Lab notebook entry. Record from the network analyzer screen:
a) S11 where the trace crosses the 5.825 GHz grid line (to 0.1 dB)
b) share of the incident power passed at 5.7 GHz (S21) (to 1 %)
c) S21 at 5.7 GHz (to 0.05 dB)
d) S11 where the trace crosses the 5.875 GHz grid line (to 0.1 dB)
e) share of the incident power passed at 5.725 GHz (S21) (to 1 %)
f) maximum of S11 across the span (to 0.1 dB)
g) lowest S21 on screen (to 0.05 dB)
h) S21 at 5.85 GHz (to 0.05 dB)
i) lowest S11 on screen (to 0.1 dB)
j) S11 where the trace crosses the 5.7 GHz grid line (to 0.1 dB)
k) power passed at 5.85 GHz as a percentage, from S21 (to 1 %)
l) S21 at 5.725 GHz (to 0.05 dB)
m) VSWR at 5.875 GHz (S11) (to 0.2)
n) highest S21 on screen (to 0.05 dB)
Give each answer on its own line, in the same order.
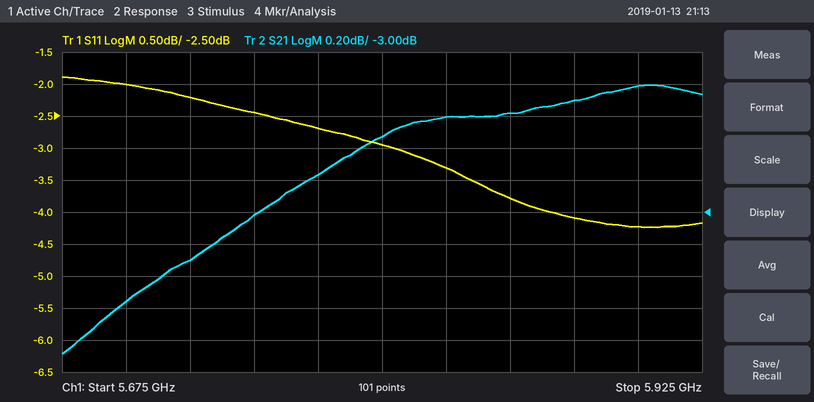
-3.3 dB
44 %
-3.55 dB
-4.1 dB
47 %
-1.9 dB
-3.90 dB
-2.40 dB
-4.2 dB
-2.0 dB
58 %
-3.30 dB
4.4
-2.20 dB
